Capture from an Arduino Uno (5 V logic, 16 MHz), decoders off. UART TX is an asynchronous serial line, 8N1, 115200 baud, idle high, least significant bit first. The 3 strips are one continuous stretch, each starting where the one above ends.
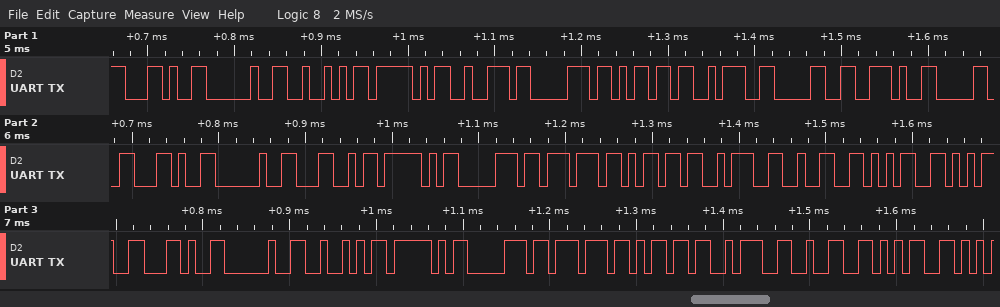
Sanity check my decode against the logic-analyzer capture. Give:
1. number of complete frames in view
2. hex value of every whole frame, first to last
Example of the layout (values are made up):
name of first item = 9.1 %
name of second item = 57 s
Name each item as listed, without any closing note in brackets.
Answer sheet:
number of complete frames in view = 32
hex value of every whole frame, first to last = 2C 20 52 5F 72 70 6D 3A 30 2E 30 2C 20 4C 5F 70 77 6D 3A 32 35 35 2C 20 52 5F 70 77 6D 3A 32 35
